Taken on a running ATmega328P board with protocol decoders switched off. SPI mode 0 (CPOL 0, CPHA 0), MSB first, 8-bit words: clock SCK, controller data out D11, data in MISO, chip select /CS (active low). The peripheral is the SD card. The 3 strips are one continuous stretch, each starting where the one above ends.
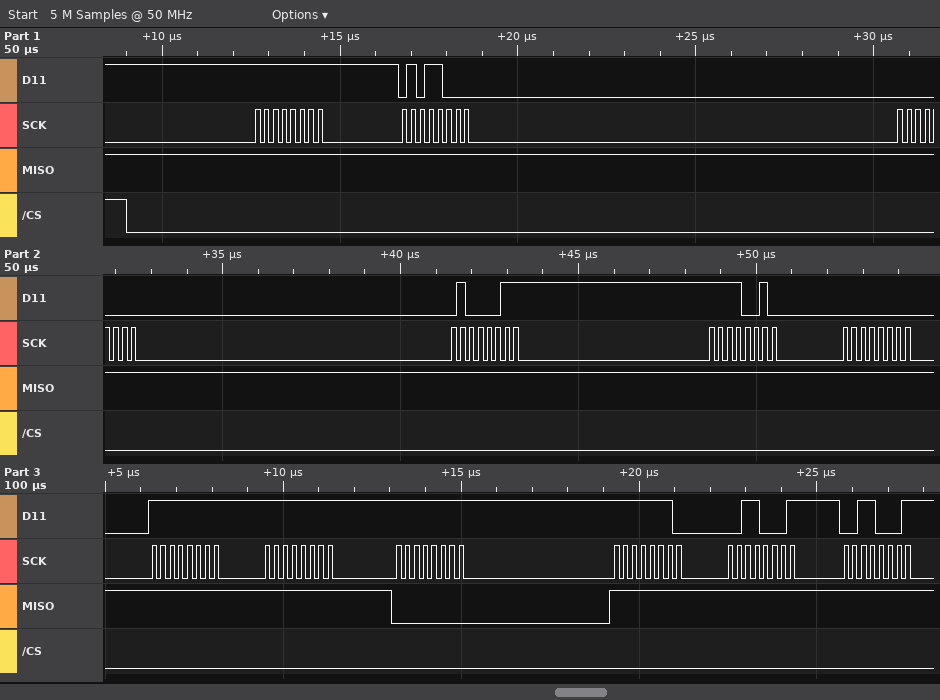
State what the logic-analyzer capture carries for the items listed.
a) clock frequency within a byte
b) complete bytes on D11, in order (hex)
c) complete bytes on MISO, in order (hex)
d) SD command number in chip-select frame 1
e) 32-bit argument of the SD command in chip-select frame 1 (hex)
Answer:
4 MHz
FF 58 00 43 F2 00 FF FF FF FE 31 31
FF FF FF FF FF FF FF FF 00 FF FF FF
CMD24
0x0043F200
